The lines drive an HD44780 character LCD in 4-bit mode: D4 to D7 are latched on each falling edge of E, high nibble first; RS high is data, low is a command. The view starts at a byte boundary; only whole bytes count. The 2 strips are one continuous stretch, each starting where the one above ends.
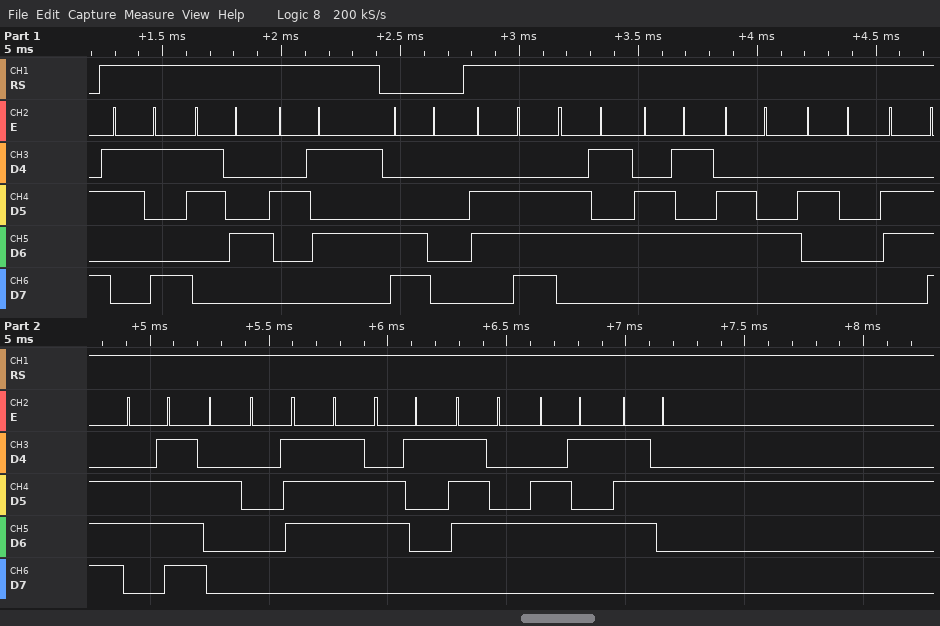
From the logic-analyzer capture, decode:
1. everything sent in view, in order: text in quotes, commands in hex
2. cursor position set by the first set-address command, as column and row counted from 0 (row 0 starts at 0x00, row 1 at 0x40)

"94%" 0xC0 "need no water"
column 0, row 1
